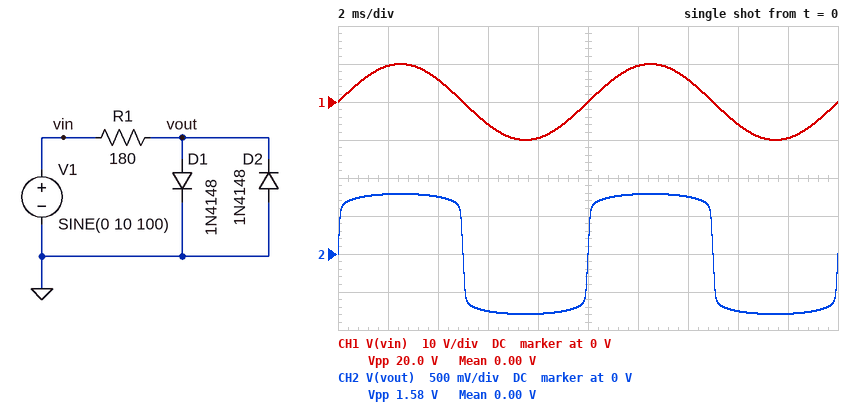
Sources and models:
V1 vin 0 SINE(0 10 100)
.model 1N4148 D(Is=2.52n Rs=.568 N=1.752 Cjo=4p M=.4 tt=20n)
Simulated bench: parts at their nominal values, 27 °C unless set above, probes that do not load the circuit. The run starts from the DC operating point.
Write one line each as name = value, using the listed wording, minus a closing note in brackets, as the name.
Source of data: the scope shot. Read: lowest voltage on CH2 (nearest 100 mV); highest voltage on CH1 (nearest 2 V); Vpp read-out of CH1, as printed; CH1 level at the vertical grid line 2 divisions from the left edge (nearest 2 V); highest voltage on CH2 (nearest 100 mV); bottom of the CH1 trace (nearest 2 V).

lowest voltage on CH2 = -800 mV
highest voltage on CH1 = 10 V
Vpp read-out of CH1, as printed = 20.0 V
CH1 level at the vertical grid line 2 divisions from the left edge = 6 V
highest voltage on CH2 = 800 mV
bottom of the CH1 trace = -10 V
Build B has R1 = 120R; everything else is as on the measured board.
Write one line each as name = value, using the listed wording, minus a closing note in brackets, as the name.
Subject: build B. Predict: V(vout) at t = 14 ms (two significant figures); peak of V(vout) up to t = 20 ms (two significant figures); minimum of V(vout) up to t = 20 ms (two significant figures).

V(vout) at t = 14 ms = 780 mV
peak of V(vout) up to t = 20 ms = 820 mV
minimum of V(vout) up to t = 20 ms = -820 mV
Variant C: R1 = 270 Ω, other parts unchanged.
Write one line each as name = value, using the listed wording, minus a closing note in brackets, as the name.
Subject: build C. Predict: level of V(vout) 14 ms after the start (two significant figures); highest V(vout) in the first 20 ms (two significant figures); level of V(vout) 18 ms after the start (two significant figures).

level of V(vout) 14 ms after the start = 730 mV
highest V(vout) in the first 20 ms = 760 mV
level of V(vout) 18 ms after the start = -760 mV
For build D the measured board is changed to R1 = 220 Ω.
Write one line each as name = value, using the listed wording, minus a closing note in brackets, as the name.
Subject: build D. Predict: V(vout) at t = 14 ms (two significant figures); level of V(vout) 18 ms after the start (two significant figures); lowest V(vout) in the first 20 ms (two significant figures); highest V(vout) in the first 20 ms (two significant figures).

V(vout) at t = 14 ms = 740 mV
level of V(vout) 18 ms after the start = -770 mV
lowest V(vout) in the first 20 ms = -780 mV
highest V(vout) in the first 20 ms = 780 mV
